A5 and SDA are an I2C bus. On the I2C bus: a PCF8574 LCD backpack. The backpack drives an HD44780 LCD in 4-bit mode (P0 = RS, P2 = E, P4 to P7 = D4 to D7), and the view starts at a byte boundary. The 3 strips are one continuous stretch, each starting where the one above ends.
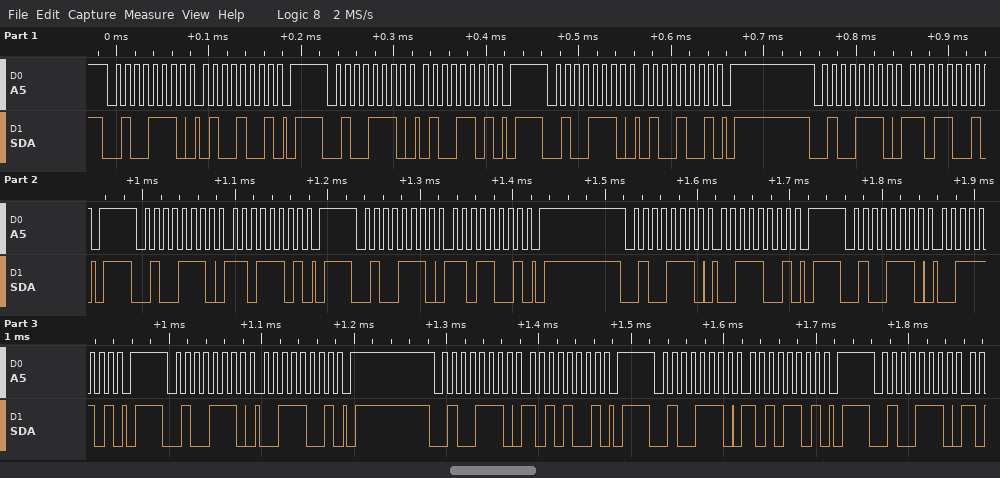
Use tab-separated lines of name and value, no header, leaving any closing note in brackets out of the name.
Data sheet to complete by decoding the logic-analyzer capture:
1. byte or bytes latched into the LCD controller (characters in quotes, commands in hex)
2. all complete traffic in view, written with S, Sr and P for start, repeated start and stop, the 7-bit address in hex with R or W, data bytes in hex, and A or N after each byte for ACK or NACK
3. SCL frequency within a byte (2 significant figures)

byte or bytes latched into the LCD controller	'M'
all complete traffic in view, written with S, Sr and P for start, repeated start and stop, the 7-bit address in hex with R or W, data bytes in hex, and A or N after each byte for ACK or NACK	S 27W A 49 A P S 27W A 4D A P S 27W A 49 A P S 27W A D9 A P S 27W A DD A P S 27W A D9 A P S 27W A 39 A P S 27W A 3D A P S 27W A 39 A P S 27W A A9 A P S 27W A AD A P S 27W A
SCL frequency within a byte	100 kHz
